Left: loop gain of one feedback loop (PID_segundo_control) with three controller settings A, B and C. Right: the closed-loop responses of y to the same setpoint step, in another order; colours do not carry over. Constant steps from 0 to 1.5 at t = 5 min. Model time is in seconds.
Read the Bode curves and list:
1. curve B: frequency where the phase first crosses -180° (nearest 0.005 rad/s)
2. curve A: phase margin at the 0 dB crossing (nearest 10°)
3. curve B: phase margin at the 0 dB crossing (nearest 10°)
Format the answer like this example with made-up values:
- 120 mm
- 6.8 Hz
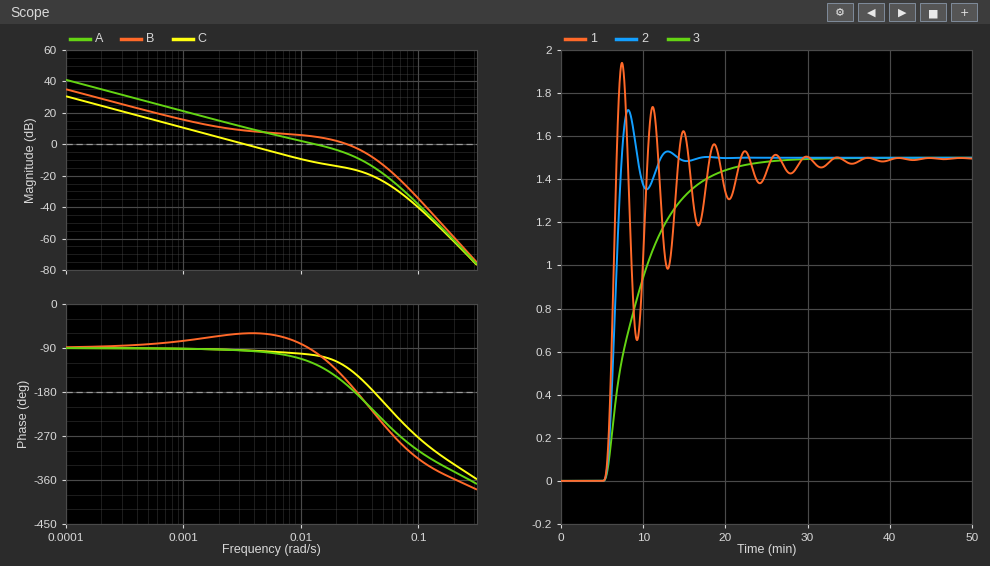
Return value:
- 0.030 rad/s
- 60°
- 20°
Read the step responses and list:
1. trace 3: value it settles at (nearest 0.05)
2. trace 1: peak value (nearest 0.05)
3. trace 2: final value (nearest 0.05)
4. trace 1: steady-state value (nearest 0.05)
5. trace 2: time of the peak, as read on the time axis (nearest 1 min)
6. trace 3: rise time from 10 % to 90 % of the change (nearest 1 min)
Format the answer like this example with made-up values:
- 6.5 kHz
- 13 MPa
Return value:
- 1.50
- 1.95
- 1.50
- 1.50
- 8 min
- 10 min
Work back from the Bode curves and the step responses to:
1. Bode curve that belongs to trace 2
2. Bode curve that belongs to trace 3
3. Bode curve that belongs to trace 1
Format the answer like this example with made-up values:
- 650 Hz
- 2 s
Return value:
- A
- C
- B
